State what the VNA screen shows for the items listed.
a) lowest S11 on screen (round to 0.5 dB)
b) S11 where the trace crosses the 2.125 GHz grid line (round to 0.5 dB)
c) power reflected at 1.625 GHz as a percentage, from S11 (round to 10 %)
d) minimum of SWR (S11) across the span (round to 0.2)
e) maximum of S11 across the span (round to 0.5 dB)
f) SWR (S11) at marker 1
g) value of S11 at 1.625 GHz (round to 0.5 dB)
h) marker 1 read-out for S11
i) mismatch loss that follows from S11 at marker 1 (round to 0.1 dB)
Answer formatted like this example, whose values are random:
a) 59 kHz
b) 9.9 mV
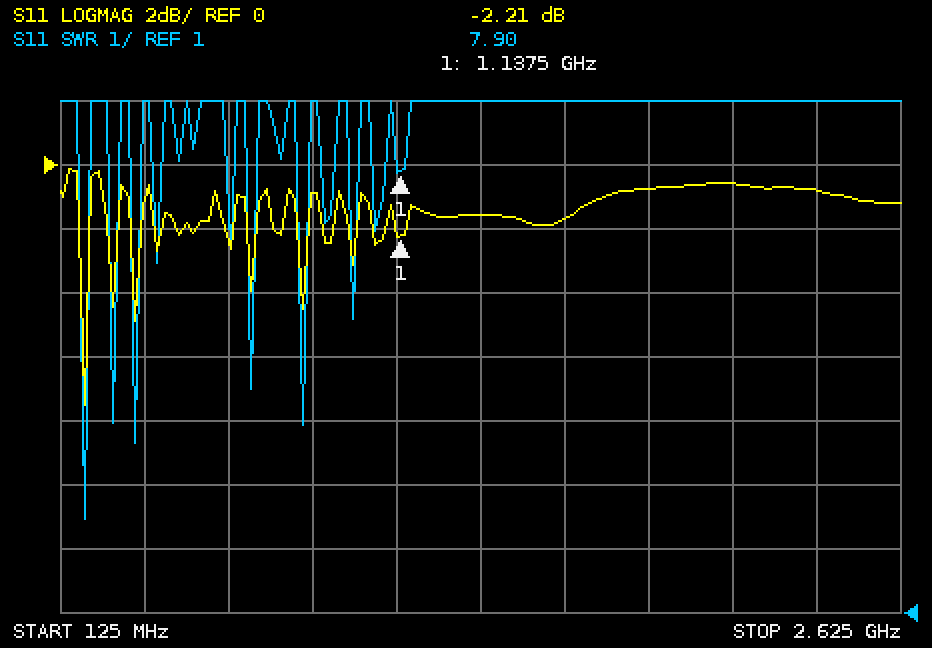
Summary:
a) -7.5 dB
b) -0.5 dB
c) 70 %
d) 2.4
e) 0.0 dB
f) 7.90
g) -1.5 dB
h) -2.21 dB
i) 4.0 dB
